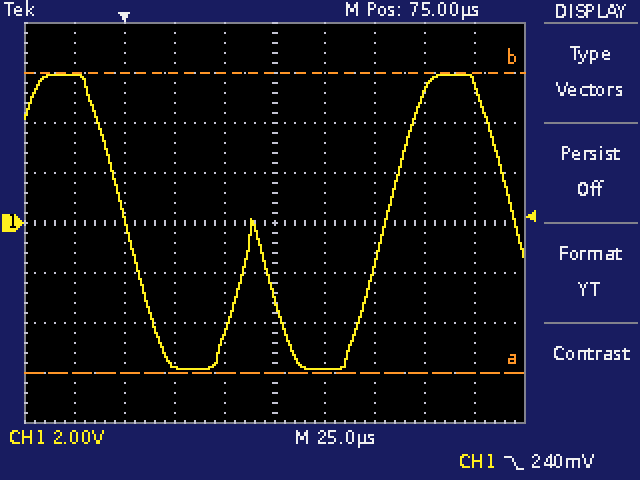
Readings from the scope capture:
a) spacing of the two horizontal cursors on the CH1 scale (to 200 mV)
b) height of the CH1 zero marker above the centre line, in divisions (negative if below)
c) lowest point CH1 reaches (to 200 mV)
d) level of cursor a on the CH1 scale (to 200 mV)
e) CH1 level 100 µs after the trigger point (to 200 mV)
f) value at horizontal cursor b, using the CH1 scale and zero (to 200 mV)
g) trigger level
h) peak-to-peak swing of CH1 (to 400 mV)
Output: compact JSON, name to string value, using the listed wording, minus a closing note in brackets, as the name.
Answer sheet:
{"spacing of the two horizontal cursors on the CH1 scale": "12.0 V", "height of the CH1 zero marker above the centre line, in divisions": "0.0 div", "lowest point CH1 reaches": "-5.8 V", "level of cursor a on the CH1 scale": "-6.0 V", "CH1 level 100 µs after the trigger point": "-5.8 V", "value at horizontal cursor b, using the CH1 scale and zero": "6.0 V", "trigger level": "240 mV", "peak-to-peak swing of CH1": "11.6 V"}
